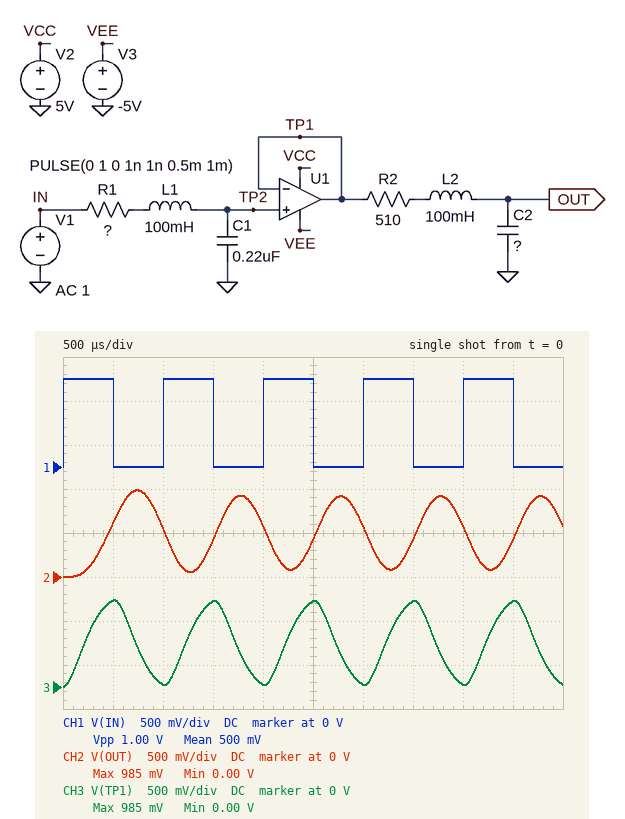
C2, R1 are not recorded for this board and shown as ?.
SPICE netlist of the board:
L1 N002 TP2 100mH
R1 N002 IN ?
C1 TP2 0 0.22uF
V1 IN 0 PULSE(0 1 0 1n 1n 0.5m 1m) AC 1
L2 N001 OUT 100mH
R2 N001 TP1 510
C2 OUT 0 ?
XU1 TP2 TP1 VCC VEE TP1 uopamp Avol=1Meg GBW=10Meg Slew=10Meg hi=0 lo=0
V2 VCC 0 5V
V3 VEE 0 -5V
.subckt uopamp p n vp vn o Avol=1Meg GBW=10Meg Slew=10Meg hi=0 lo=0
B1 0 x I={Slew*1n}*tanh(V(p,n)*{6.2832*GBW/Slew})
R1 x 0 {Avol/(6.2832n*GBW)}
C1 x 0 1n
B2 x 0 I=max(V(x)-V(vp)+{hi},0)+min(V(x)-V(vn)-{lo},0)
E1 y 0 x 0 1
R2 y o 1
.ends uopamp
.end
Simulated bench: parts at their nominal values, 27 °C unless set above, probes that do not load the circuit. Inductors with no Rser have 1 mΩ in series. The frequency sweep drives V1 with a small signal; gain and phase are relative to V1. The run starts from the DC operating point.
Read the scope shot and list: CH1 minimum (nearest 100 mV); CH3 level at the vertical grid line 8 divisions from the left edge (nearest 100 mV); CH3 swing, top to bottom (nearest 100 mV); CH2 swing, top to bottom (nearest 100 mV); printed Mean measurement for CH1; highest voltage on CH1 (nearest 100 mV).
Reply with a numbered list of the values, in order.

1. 0 V
2. 0 V
3. 1.0 V
4. 1.0 V
5. 500 mV
6. 1.0 V
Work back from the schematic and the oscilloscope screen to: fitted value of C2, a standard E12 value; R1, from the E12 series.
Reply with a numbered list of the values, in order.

1. 330 nF
2. 1 kΩ
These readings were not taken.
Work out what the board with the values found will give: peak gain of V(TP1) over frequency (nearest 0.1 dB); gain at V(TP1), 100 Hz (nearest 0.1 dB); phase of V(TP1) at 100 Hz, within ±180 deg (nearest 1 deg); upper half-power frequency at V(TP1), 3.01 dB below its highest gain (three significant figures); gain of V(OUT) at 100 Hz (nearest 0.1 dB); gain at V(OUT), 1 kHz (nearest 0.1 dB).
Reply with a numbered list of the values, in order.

1. 0 dB
2. 0 dB
3. -8 deg
4. 1.02 kHz
5. 0.1 dB
6. -3.7 dB
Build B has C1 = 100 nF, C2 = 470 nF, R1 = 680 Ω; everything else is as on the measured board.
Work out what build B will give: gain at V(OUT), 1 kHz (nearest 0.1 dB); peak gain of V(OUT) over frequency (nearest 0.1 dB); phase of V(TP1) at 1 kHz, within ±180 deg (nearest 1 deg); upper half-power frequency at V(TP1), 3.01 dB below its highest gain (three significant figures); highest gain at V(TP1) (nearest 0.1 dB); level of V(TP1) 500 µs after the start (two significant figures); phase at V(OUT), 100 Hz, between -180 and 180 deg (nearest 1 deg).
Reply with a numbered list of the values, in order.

1. -2.2 dB
2. 1.4 dB
3. -35 deg
4. 1.89 kHz
5. 3.9 dB
6. 1.1 V
7. -11 deg
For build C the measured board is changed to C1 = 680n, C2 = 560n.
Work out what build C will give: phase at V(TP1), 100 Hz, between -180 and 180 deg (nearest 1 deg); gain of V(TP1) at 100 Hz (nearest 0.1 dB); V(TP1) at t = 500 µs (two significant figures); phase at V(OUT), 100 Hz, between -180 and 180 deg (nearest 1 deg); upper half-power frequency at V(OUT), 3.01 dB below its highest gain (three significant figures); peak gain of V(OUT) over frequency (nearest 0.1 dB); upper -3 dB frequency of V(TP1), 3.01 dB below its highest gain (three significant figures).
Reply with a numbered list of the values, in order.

1. -24 deg
2. -0.5 dB
3. 480 mV
4. -34 deg
5. 291 Hz
6. 0 dB
7. 273 Hz
